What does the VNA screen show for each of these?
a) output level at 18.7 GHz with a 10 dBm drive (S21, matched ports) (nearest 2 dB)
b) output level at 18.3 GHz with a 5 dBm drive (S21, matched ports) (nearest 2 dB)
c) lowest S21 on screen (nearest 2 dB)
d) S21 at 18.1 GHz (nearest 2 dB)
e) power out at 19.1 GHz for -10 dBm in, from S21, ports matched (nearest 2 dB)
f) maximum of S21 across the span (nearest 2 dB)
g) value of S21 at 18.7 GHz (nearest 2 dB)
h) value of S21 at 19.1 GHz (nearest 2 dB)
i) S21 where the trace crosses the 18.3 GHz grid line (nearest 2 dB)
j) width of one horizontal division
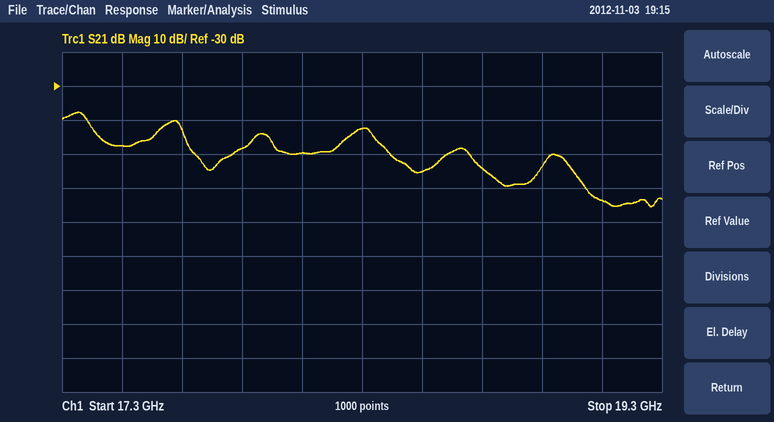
-44 dBm
-38 dBm
-66 dB
-50 dB
-74 dBm
-38 dB
-54 dB
-64 dB
-42 dB
200 MHz
